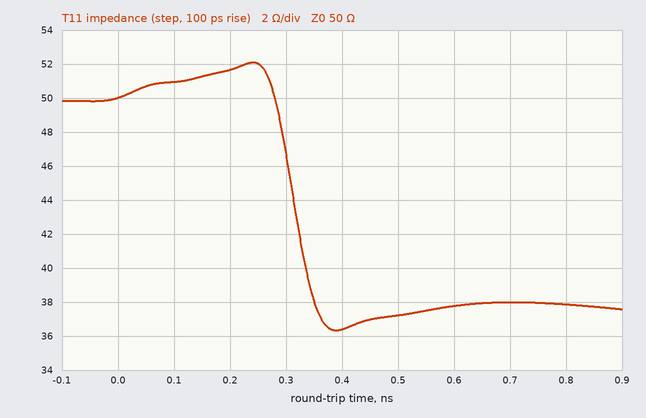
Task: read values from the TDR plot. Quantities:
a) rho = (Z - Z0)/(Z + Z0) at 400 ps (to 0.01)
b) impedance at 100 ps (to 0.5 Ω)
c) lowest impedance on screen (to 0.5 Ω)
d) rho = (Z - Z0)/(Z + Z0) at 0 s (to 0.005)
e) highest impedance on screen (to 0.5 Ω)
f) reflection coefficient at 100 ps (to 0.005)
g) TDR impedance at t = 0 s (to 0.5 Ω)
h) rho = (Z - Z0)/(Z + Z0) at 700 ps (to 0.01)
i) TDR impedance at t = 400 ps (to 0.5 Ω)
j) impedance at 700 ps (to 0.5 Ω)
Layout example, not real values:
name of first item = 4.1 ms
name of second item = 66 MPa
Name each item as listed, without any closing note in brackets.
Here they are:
rho = (Z - Z0)/(Z + Z0) at 400 ps = -0.16
impedance at 100 ps = 51.0 Ω
lowest impedance on screen = 36.5 Ω
rho = (Z - Z0)/(Z + Z0) at 0 s = 0.000
highest impedance on screen = 52.0 Ω
reflection coefficient at 100 ps = +0.010
TDR impedance at t = 0 s = 50.0 Ω
rho = (Z - Z0)/(Z + Z0) at 700 ps = -0.14
TDR impedance at t = 400 ps = 36.5 Ω
impedance at 700 ps = 38.0 Ω
